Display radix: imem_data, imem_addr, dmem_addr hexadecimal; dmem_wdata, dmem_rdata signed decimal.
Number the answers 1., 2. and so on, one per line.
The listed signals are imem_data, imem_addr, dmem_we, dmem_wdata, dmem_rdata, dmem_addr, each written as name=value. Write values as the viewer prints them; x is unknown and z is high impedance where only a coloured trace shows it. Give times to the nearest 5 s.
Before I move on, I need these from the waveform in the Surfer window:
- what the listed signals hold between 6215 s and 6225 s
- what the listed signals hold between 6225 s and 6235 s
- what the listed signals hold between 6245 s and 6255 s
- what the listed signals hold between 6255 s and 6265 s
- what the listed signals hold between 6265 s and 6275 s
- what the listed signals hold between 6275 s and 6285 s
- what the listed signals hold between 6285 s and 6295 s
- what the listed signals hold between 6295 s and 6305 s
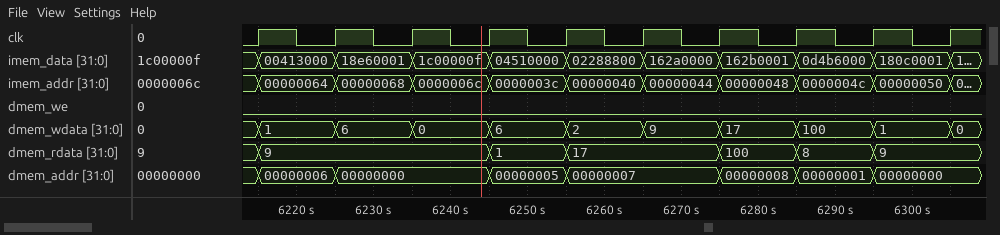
1. imem_data=00413000, imem_addr=00000064, dmem_we=0, dmem_wdata=1, dmem_rdata=9, dmem_addr=00000006
2. imem_data=18e60001, imem_addr=00000068, dmem_we=0, dmem_wdata=6, dmem_rdata=9, dmem_addr=00000000
3. imem_data=04510000, imem_addr=0000003c, dmem_we=0, dmem_wdata=6, dmem_rdata=1, dmem_addr=00000005
4. imem_data=02288800, imem_addr=00000040, dmem_we=0, dmem_wdata=2, dmem_rdata=17, dmem_addr=00000007
5. imem_data=162a0000, imem_addr=00000044, dmem_we=0, dmem_wdata=9, dmem_rdata=17, dmem_addr=00000007
6. imem_data=162b0001, imem_addr=00000048, dmem_we=0, dmem_wdata=17, dmem_rdata=100, dmem_addr=00000008
7. imem_data=0d4b6000, imem_addr=0000004c, dmem_we=0, dmem_wdata=100, dmem_rdata=8, dmem_addr=00000001
8. imem_data=180c0001, imem_addr=00000050, dmem_we=0, dmem_wdata=1, dmem_rdata=9, dmem_addr=00000000
